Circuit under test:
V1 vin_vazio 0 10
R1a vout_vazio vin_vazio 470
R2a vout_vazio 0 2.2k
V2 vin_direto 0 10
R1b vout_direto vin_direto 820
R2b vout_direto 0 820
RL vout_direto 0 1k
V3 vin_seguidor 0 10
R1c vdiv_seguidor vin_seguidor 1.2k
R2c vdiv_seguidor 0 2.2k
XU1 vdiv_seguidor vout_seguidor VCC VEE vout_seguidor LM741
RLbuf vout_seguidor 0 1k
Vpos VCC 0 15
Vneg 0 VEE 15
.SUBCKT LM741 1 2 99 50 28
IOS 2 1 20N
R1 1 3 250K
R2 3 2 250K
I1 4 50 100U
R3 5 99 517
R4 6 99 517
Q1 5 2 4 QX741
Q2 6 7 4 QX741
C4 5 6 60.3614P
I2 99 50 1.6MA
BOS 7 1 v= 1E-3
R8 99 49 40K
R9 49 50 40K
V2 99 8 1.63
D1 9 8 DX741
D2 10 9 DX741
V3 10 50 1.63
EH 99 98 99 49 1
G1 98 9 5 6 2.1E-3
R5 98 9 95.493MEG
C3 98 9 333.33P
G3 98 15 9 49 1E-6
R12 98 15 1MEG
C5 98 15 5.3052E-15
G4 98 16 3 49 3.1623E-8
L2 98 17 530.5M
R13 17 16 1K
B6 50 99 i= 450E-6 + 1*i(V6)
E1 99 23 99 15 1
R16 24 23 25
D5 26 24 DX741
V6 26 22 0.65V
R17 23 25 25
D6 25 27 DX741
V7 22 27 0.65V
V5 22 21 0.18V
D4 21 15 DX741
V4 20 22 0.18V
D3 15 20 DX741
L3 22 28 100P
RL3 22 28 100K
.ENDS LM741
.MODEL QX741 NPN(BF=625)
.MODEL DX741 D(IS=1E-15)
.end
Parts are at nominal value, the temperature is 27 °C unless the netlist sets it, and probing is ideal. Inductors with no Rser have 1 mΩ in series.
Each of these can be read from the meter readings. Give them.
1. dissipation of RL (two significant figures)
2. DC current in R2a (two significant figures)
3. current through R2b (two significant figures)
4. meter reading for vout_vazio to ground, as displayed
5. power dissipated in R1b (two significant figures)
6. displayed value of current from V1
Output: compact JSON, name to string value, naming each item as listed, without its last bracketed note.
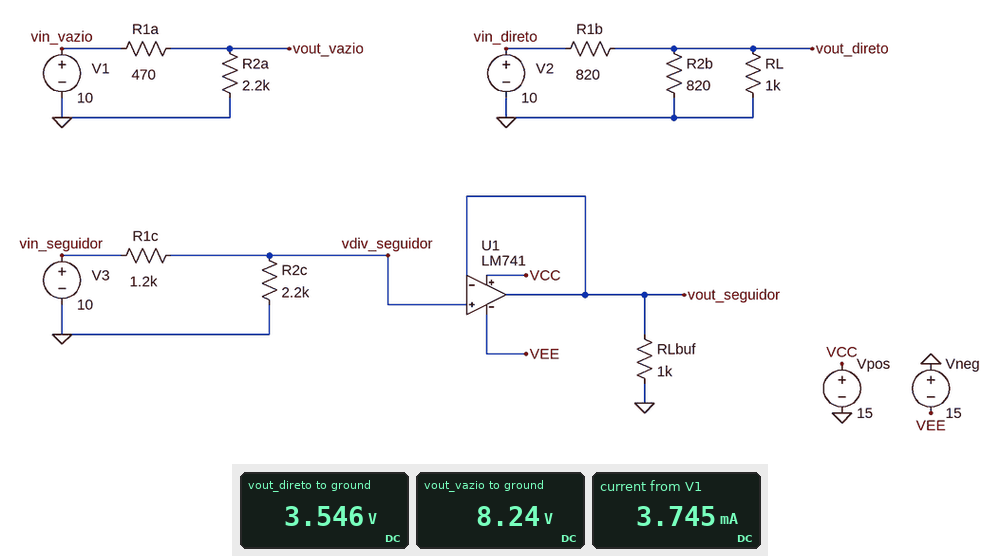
{"dissipation of RL": "13 mW", "DC current in R2a": "3.7 mA", "current through R2b": "4.3 mA", "meter reading for vout_vazio to ground, as displayed": "8.24 V", "power dissipated in R1b": "51 mW", "displayed value of current from V1": "3.745 mA"}
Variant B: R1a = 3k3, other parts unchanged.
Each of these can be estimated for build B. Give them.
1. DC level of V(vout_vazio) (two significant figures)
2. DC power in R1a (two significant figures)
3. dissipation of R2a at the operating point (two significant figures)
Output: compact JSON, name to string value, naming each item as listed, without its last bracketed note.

{"DC level of V(vout_vazio)": "4.0 V", "DC power in R1a": "11 mW", "dissipation of R2a at the operating point": "7.3 mW"}
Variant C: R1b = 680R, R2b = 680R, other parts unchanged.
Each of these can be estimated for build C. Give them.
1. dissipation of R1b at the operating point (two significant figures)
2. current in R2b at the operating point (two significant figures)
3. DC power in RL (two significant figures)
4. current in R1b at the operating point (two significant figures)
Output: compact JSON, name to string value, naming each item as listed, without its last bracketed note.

{"dissipation of R1b at the operating point": "58 mW", "current in R2b at the operating point": "5.5 mA", "DC power in RL": "14 mW", "current in R1b at the operating point": "9.2 mA"}
